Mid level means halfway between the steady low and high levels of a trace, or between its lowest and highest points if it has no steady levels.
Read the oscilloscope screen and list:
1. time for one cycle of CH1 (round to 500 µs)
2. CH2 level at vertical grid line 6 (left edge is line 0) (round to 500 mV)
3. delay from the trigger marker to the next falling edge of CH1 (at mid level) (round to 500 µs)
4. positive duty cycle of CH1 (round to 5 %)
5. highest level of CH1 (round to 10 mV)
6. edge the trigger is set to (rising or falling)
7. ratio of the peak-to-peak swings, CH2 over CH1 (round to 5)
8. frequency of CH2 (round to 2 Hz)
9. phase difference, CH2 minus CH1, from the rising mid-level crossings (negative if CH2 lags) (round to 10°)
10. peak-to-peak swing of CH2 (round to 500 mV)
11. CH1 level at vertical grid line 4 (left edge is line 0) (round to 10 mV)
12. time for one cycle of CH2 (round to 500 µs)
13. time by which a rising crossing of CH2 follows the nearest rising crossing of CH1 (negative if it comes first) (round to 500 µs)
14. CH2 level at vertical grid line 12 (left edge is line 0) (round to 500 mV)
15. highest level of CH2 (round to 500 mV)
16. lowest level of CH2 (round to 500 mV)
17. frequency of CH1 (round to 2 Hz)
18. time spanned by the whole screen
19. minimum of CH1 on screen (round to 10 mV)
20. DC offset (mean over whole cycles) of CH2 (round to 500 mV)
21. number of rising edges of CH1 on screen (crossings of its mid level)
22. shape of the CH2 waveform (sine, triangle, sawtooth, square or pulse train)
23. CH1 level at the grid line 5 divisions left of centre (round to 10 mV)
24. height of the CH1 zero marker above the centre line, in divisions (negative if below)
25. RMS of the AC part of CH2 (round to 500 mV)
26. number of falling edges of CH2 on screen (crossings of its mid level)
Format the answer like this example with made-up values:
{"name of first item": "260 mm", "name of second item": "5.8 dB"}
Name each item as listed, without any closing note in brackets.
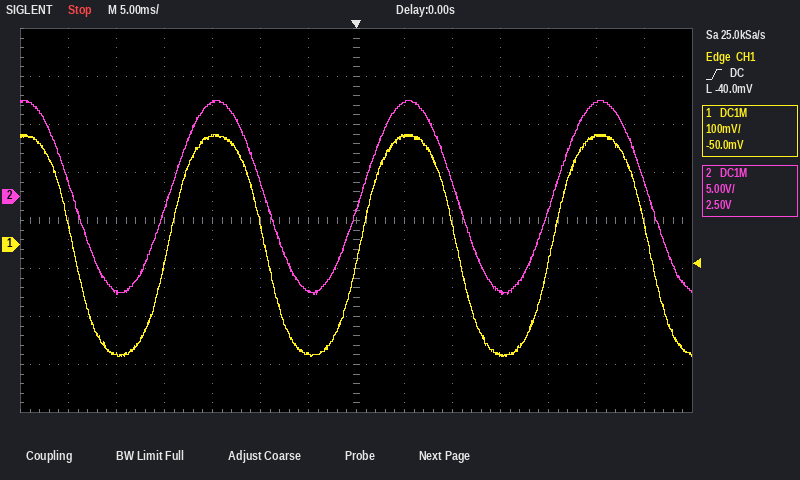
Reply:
{"time for one cycle of CH1": "20.0 ms", "CH2 level at vertical grid line 6 (left edge is line 0)": "-10.0 V", "delay from the trigger marker to the next falling edge of CH1 (at mid level)": "10.5 ms", "positive duty cycle of CH1": "50 %", "highest level of CH1": "230 mV", "edge the trigger is set to": "rising", "ratio of the peak-to-peak swings, CH2 over CH1": "45", "frequency of CH2": "50 Hz", "phase difference, CH2 minus CH1, from the rising mid-level crossings (negative if CH2 lags)": "0°", "peak-to-peak swing of CH2": "20.0 V", "CH1 level at vertical grid line 4 (left edge is line 0)": "230 mV", "time for one cycle of CH2": "20.0 ms", "time by which a rising crossing of CH2 follows the nearest rising crossing of CH1 (negative if it comes first)": "0.0 ms", "CH2 level at vertical grid line 12 (left edge is line 0)": "10.0 V", "highest level of CH2": "10.0 V", "lowest level of CH2": "-10.0 V", "frequency of CH1": "50 Hz", "time spanned by the whole screen": "70 ms", "minimum of CH1 on screen": "-230 mV", "DC offset (mean over whole cycles) of CH2": "0.0 V", "number of rising edges of CH1 on screen": "3", "shape of the CH2 waveform": "sine", "CH1 level at the grid line 5 divisions left of centre": "-230 mV", "height of the CH1 zero marker above the centre line, in divisions": "-0.5 div", "RMS of the AC part of CH2": "7.0 V", "number of falling edges of CH2 on screen": "4"}
